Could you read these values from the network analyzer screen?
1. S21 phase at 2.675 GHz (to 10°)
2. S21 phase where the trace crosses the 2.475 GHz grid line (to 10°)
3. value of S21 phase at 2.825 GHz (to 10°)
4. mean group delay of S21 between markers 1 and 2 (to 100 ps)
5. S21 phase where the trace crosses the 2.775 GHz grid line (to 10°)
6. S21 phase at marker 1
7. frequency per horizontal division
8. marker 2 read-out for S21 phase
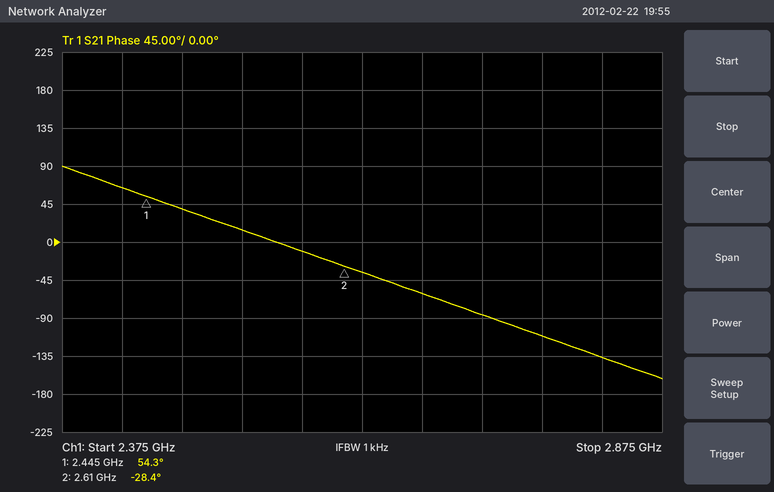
-60°
40°
-140°
1.4 ns
-110°
54.3°
50 MHz
-28.4°
